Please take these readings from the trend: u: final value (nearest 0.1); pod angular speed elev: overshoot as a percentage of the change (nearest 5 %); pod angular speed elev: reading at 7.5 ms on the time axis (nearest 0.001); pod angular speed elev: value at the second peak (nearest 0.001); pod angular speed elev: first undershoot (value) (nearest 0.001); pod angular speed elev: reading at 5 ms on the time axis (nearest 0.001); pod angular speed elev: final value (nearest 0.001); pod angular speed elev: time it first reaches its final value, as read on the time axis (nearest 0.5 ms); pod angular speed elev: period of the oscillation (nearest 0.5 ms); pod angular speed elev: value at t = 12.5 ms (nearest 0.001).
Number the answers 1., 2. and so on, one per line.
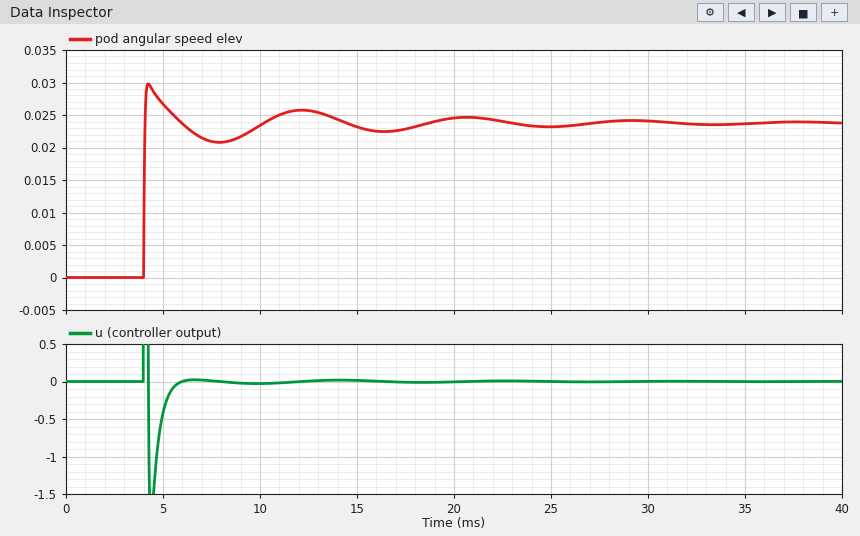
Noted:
1. 0.0
2. 25 %
3. 0.021
4. 0.026
5. 0.021
6. 0.027
7. 0.024
8. 4.0 ms
9. 8.0 ms
10. 0.026
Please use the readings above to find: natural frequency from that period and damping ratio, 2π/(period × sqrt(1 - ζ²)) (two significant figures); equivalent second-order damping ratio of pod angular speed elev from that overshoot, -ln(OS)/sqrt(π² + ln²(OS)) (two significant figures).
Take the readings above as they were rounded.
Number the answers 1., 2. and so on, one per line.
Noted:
1. 0.86 rad/ms
2. 0.40
